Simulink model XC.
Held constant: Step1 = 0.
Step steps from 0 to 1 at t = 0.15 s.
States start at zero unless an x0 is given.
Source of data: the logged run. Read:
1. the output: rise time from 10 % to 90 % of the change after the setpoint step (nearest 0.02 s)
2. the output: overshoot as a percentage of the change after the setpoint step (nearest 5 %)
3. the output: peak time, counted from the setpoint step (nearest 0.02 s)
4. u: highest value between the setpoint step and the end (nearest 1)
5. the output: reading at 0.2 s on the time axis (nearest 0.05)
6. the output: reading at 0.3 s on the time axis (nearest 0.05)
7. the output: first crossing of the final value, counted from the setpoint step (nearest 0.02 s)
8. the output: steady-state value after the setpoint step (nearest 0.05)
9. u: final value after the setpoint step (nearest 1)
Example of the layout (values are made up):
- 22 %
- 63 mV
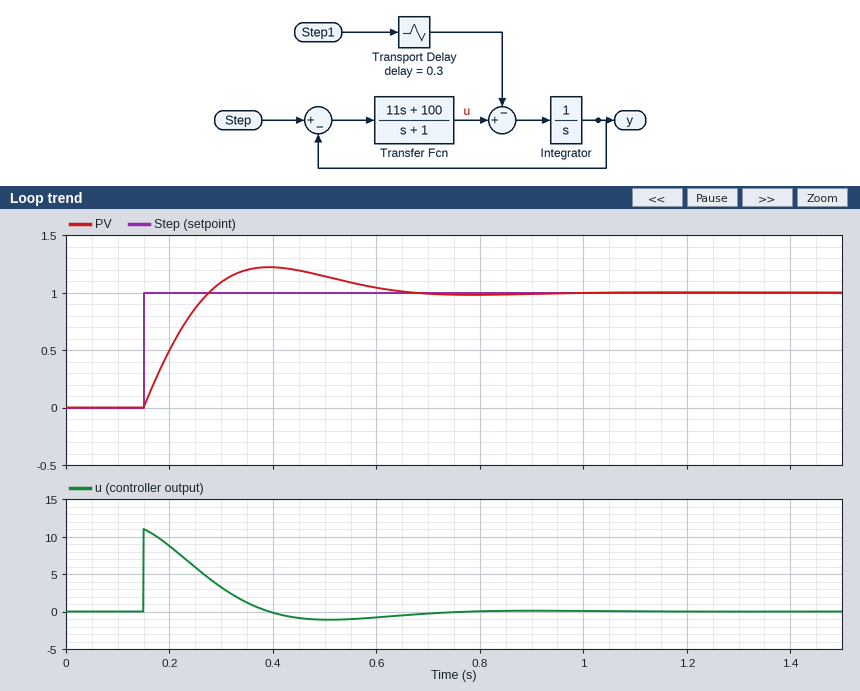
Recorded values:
- 0.10 s
- 20 %
- 0.24 s
- 11
- 0.50
- 1.10
- 0.12 s
- 1.00
- 0
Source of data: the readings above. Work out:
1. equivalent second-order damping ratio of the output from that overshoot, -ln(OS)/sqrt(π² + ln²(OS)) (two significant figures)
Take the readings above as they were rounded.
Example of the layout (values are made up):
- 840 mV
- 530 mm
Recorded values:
- 0.46
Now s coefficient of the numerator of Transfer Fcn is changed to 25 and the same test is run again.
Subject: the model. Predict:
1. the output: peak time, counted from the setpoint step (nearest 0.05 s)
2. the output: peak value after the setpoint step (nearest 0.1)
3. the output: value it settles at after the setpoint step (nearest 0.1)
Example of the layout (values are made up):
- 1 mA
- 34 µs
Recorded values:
- 0.20 s
- 1.1
- 1.0
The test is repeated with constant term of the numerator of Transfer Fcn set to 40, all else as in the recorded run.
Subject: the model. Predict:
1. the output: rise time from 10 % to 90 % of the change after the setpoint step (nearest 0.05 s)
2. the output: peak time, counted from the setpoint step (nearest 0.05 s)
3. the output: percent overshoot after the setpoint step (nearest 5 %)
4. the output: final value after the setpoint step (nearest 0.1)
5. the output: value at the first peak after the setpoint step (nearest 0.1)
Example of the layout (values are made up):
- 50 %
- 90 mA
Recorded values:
- 0.15 s
- 0.35 s
- 10 %
- 1.0
- 1.1
